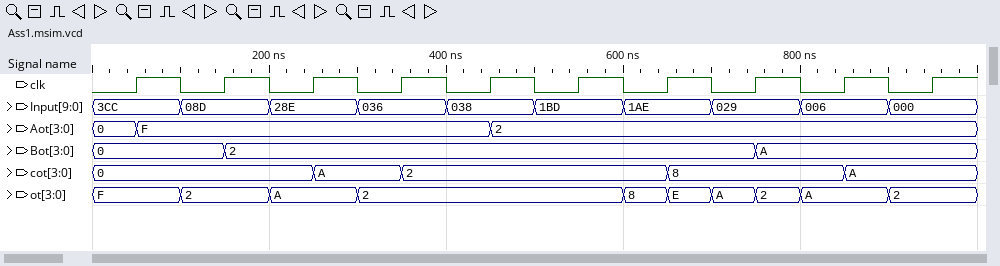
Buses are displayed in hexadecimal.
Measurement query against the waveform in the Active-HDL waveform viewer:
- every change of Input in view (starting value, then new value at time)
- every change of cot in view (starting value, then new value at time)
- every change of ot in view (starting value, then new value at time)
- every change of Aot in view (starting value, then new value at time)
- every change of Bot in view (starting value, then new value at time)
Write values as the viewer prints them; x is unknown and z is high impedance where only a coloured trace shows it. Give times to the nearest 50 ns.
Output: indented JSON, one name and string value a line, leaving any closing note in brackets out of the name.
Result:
{
  "every change of Input in view": "3CC, 08D at 100 ns, 28E at 200 ns, 036 at 300 ns, 038 at 400 ns, 1BD at 500 ns, 1AE at 600 ns, 029 at 700 ns, 006 at 800 ns, 000 at 900 ns",
  "every change of cot in view": "0, A at 250 ns, 2 at 350 ns, 8 at 650 ns, A at 850 ns",
  "every change of ot in view": "F, 2 at 100 ns, A at 200 ns, 2 at 300 ns, 8 at 600 ns, E at 650 ns, A at 700 ns, 2 at 750 ns, A at 800 ns, 2 at 900 ns",
  "every change of Aot in view": "0, F at 50 ns, 2 at 450 ns",
  "every change of Bot in view": "0, 2 at 150 ns, A at 750 ns"
}
